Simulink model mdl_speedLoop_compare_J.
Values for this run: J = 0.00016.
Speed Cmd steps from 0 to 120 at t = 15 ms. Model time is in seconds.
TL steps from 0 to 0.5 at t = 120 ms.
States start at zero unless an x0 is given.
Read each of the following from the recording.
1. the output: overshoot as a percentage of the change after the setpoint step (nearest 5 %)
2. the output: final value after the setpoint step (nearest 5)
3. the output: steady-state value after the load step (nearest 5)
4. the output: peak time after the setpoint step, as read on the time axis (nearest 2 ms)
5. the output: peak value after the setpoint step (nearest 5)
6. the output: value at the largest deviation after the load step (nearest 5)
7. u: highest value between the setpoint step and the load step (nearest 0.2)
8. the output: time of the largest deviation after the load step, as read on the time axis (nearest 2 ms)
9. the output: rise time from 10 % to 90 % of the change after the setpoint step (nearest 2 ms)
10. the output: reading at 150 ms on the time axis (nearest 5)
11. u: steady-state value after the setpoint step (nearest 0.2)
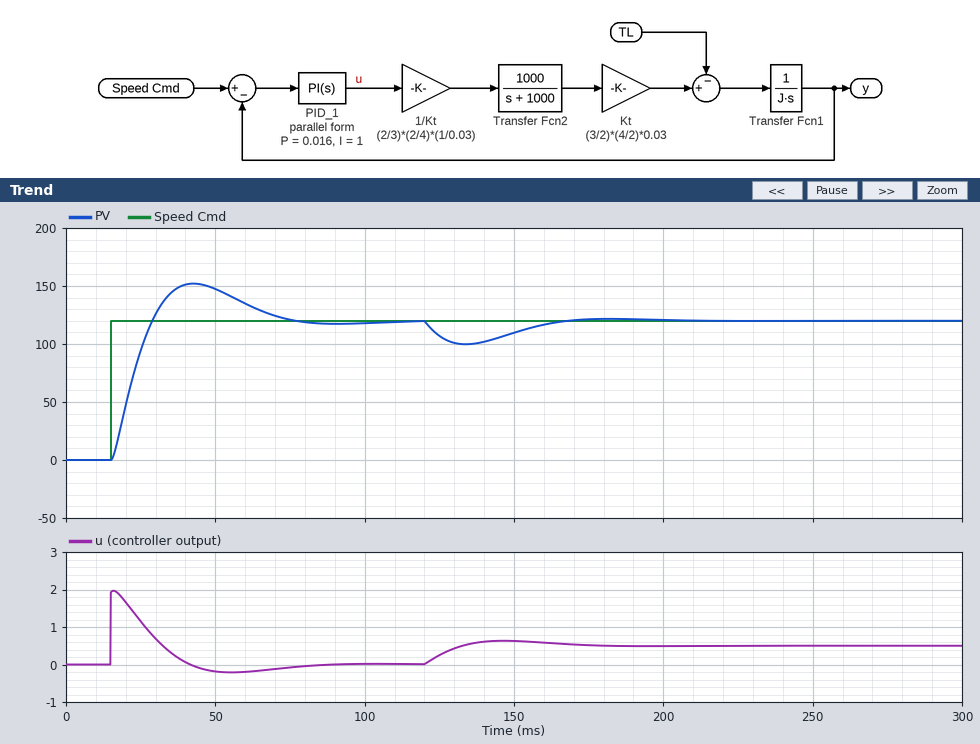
25 %
120
120
42 ms
150
100
2.0
134 ms
10 ms
110
0.0
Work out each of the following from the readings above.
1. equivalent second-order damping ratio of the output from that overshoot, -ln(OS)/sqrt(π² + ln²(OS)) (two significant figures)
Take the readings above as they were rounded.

0.40
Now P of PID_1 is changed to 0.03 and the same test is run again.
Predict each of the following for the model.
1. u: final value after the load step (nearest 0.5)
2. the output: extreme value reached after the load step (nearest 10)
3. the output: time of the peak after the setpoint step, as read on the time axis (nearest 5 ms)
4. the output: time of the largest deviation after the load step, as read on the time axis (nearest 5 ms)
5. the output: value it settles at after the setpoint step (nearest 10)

0.5
110
35 ms
130 ms
120
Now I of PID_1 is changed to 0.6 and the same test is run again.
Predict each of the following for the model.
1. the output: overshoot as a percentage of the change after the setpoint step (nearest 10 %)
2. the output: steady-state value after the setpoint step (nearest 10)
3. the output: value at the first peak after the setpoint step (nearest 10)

20 %
120
140
